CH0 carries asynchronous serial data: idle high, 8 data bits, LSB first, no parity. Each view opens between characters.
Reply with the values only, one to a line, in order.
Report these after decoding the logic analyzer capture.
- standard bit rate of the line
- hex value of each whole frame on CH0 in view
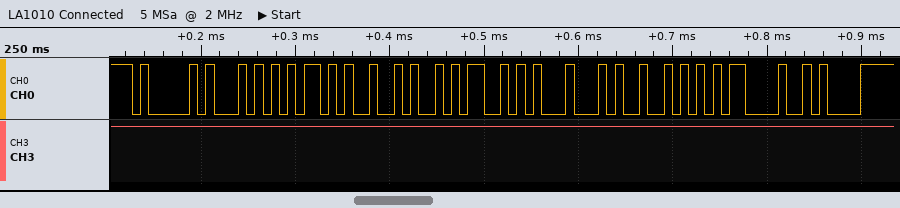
115200 baud
41, 54, 2B, 4A, 53, 44, 52, 0D, 0A
